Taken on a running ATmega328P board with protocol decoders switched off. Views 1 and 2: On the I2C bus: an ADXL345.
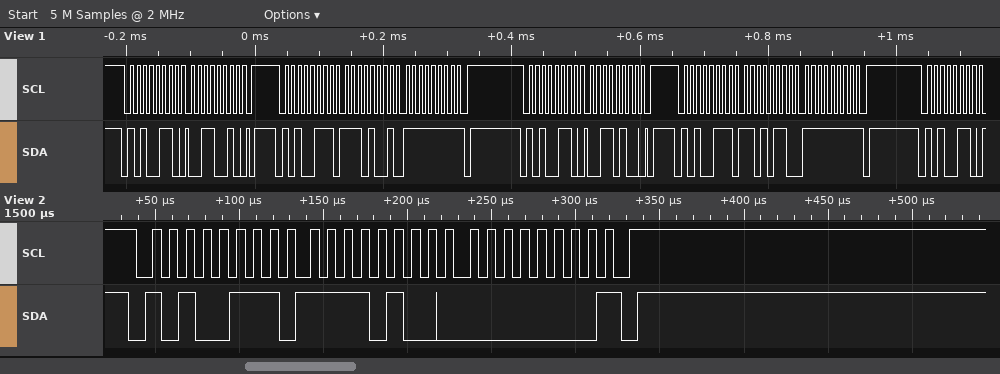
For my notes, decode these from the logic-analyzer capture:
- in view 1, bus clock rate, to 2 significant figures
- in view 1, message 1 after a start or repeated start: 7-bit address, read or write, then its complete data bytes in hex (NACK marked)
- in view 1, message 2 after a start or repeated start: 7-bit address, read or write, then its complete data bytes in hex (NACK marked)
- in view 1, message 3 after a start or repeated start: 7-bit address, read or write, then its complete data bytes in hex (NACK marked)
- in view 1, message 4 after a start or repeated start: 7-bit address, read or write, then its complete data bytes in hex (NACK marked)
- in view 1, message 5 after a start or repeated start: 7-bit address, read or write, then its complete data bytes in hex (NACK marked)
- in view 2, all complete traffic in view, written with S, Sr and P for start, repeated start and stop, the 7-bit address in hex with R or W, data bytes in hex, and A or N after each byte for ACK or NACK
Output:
100 kHz
0x53 write: 32
0x53 read: E9 FF NACK
0x53 write: 34
0x53 read: D6 FF NACK
0x53 write
S 53R A F4 A 00 N P
